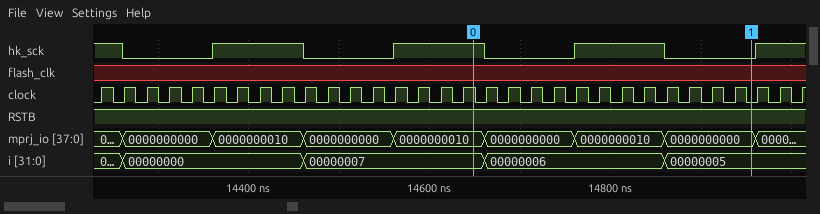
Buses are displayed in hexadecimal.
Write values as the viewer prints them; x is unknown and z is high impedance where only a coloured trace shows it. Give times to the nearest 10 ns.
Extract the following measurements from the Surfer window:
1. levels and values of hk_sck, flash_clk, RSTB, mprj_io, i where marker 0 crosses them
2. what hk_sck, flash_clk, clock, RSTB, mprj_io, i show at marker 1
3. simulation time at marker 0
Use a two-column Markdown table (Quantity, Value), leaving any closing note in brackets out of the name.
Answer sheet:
| Quantity | Value |
|---|---|
| levels and values of hk_sck, flash_clk, RSTB, mprj_io, i where marker 0 crosses them | hk_sck=1, flash_clk=x, RSTB=1, mprj_io=0000000010, i=00000007 |
| what hk_sck, flash_clk, clock, RSTB, mprj_io, i show at marker 1 | hk_sck=0, flash_clk=x, clock=0, RSTB=1, mprj_io=0000000000, i=00000005 |
| simulation time at marker 0 | 14650 ns |
